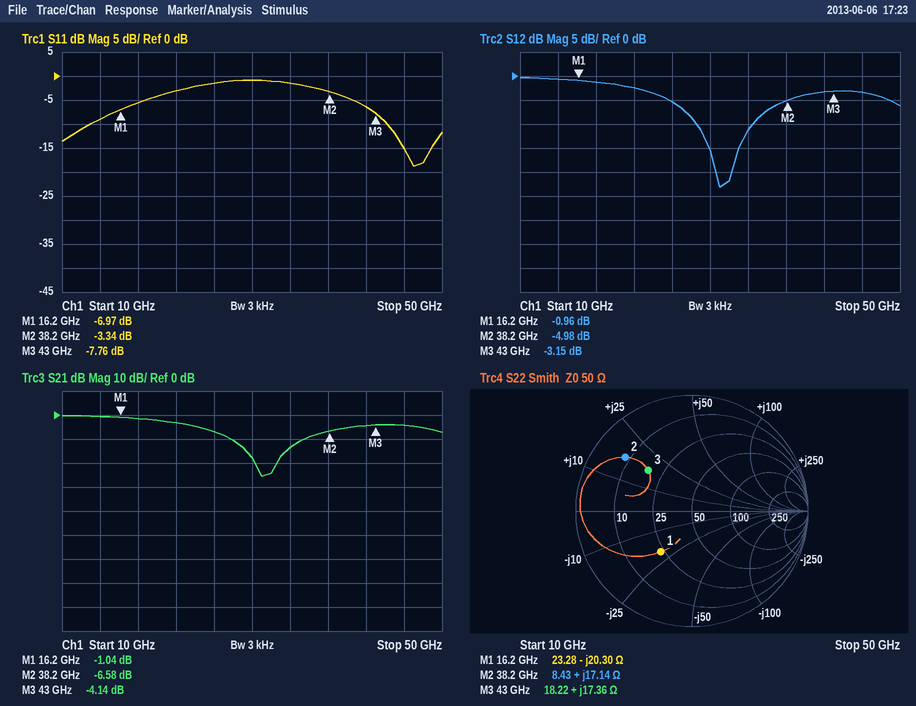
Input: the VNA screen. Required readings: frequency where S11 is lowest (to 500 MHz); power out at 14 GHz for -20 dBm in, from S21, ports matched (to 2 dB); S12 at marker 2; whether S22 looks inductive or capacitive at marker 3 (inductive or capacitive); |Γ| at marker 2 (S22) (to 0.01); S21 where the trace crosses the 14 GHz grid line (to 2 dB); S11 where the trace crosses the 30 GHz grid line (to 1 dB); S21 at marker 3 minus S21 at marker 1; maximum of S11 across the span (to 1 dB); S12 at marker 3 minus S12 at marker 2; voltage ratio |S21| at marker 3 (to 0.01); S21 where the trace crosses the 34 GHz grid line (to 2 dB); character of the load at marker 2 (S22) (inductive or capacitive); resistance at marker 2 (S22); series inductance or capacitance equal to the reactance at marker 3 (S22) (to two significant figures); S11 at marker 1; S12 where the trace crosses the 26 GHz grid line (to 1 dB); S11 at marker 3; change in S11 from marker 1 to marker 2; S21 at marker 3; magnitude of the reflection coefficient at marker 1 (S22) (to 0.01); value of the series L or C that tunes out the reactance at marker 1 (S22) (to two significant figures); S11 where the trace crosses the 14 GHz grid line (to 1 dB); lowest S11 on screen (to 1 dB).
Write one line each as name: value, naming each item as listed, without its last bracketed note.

frequency where S11 is lowest: 47.0 GHz
power out at 14 GHz for -20 dBm in, from S21, ports matched: -20 dBm
S12 at marker 2: -4.98 dB
whether S22 looks inductive or capacitive at marker 3: inductive
|Γ| at marker 2 (S22): 0.74
S21 where the trace crosses the 14 GHz grid line: 0 dB
S11 where the trace crosses the 30 GHz grid line: -1 dB
S21 at marker 3 minus S21 at marker 1: -3.10 dB
maximum of S11 across the span: -1 dB
S12 at marker 3 minus S12 at marker 2: 1.83 dB
voltage ratio |S21| at marker 3: 0.62
S21 where the trace crosses the 34 GHz grid line: -14 dB
character of the load at marker 2 (S22): inductive
resistance at marker 2: 8.43 Ω
series inductance or capacitance equal to the reactance at marker 3 (S22): 64 pH
S11 at marker 1: -6.97 dB
S12 where the trace crosses the 26 GHz grid line: -5 dB
S11 at marker 3: -7.76 dB
change in S11 from marker 1 to marker 2: 3.63 dB
S21 at marker 3: -4.14 dB
magnitude of the reflection coefficient at marker 1 (S22): 0.44
value of the series L or C that tunes out the reactance at marker 1 (S22): 200 pH
S11 where the trace crosses the 14 GHz grid line: -9 dB
lowest S11 on screen: -19 dB
